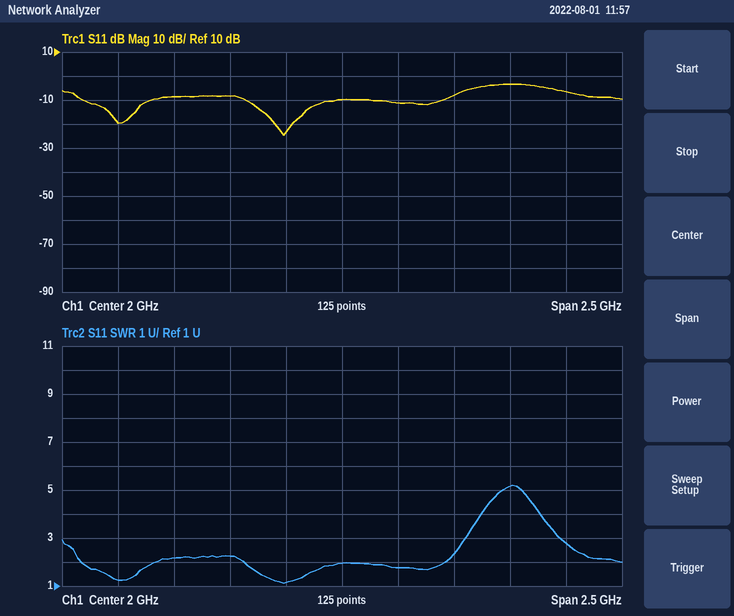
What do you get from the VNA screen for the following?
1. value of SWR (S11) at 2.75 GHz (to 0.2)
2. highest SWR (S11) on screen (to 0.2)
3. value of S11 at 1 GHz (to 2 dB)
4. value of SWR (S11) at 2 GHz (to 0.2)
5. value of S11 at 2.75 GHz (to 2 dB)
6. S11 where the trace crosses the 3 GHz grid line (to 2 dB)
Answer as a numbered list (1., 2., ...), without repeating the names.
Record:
1. 5.2
2. 5.2
3. -20 dB
4. 2.0
5. -4 dB
6. -6 dB
